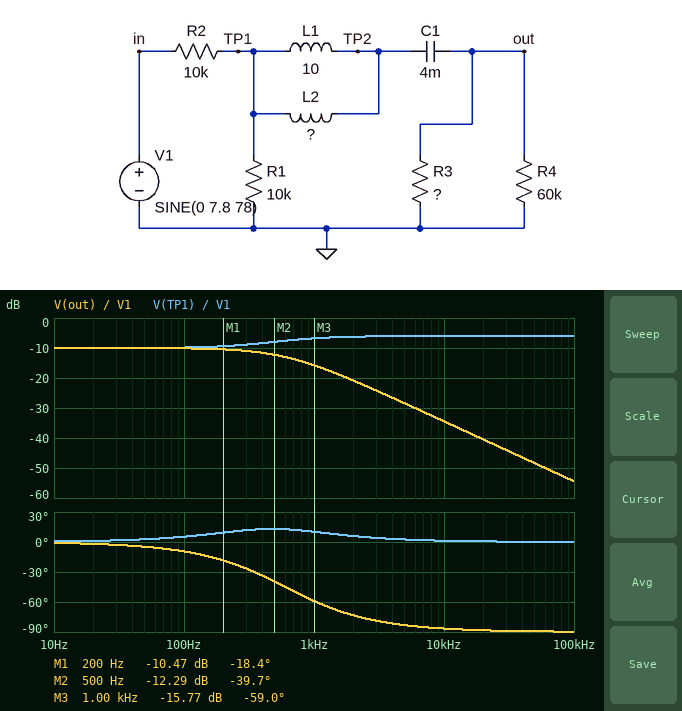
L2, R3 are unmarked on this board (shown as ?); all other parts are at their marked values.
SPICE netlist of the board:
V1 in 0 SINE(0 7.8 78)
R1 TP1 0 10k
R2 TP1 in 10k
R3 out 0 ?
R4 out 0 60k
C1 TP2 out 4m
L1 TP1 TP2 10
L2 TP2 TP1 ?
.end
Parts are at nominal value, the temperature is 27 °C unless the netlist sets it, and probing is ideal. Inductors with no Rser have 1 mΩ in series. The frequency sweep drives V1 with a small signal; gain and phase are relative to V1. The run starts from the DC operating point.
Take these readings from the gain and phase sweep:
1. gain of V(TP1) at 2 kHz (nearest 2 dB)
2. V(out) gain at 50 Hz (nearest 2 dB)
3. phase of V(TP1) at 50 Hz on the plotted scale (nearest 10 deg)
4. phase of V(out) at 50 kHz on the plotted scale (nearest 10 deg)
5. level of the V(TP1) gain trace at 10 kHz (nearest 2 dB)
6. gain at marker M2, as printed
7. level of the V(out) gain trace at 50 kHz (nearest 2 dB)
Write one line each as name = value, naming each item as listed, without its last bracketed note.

gain of V(TP1) at 2 kHz = -6 dB
V(out) gain at 50 Hz = -10 dB
phase of V(TP1) at 50 Hz on the plotted scale = 0 deg
phase of V(out) at 50 kHz on the plotted scale = -90 deg
level of the V(TP1) gain trace at 10 kHz = -6 dB
gain at marker M2, as printed = -12.29 dB
level of the V(out) gain trace at 50 kHz = -48 dB
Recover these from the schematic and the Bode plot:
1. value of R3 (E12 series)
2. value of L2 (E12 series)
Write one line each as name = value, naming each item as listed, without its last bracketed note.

value of R3 = 10 kΩ
value of L2 = 5.6 H
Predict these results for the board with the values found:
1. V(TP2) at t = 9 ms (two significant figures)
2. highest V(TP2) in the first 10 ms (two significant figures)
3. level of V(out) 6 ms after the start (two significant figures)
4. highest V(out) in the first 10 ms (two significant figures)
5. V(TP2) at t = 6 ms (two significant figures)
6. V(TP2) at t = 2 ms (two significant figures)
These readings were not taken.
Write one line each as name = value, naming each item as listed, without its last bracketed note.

V(TP2) at t = 9 ms = -2.2 V
highest V(TP2) in the first 10 ms = 2.4 V
level of V(out) 6 ms after the start = 790 mV
highest V(out) in the first 10 ms = 2.4 V
V(TP2) at t = 6 ms = 790 mV
V(TP2) at t = 2 ms = 1.8 V
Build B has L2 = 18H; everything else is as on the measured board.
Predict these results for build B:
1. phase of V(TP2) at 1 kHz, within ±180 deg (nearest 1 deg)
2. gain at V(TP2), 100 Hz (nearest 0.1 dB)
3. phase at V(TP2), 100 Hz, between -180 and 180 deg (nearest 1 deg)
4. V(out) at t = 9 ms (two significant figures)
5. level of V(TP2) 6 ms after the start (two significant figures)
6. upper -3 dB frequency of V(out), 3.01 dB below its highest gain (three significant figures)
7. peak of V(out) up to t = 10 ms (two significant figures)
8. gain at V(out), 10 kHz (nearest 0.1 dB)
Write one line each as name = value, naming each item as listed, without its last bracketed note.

phase of V(TP2) at 1 kHz, within ±180 deg = -71 deg
gain at V(TP2), 100 Hz = -10.4 dB
phase at V(TP2), 100 Hz, between -180 and 180 deg = -17 deg
V(out) at t = 9 ms = -2.1 V
level of V(TP2) 6 ms after the start = 1.0 V
upper -3 dB frequency of V(out), 3.01 dB below its highest gain = 336 Hz
peak of V(out) up to t = 10 ms = 2.4 V
gain at V(out), 10 kHz = -39.5 dB
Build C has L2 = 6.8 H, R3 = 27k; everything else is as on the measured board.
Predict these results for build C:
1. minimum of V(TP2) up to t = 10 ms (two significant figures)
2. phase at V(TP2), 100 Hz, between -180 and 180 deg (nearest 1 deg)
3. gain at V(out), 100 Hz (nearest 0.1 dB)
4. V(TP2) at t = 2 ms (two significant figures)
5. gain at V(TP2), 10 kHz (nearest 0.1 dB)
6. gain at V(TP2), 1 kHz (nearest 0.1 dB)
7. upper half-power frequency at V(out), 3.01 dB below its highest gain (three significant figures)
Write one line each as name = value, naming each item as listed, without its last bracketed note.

minimum of V(TP2) up to t = 10 ms = -3.1 V
phase at V(TP2), 100 Hz, between -180 and 180 deg = -6 deg
gain at V(out), 100 Hz = -8.1 dB
V(TP2) at t = 2 ms = 2.4 V
gain at V(TP2), 10 kHz = -28.8 dB
gain at V(TP2), 1 kHz = -11.4 dB
upper half-power frequency at V(out), 3.01 dB below its highest gain = 929 Hz
